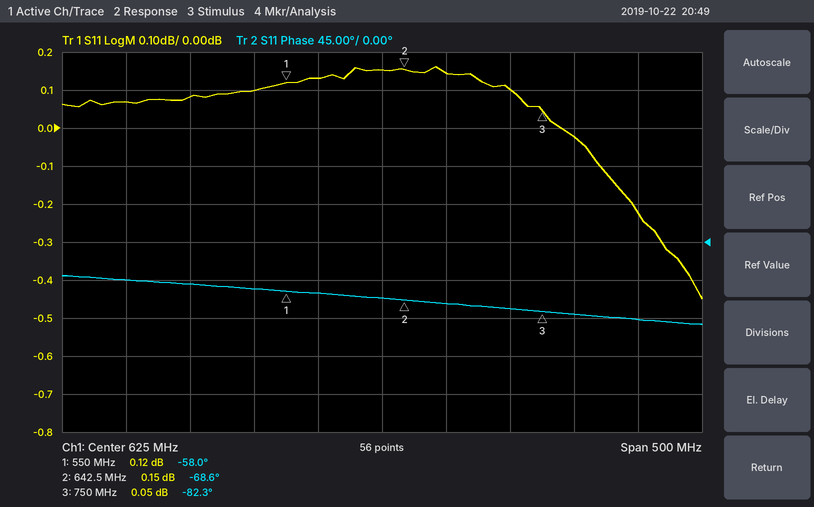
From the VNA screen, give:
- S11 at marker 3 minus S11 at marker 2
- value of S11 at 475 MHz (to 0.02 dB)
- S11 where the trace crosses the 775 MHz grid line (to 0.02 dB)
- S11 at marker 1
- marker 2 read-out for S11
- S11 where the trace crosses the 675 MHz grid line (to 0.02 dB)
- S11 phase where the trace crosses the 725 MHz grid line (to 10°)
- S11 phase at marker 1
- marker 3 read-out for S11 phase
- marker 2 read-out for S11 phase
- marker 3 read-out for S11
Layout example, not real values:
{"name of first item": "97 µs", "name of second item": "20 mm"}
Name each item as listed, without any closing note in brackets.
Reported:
{"S11 at marker 3 minus S11 at marker 2": "-0.10 dB", "value of S11 at 475 MHz": "0.08 dB", "S11 where the trace crosses the 775 MHz grid line": "-0.02 dB", "S11 at marker 1": "0.12 dB", "marker 2 read-out for S11": "0.15 dB", "S11 where the trace crosses the 675 MHz grid line": "0.14 dB", "S11 phase where the trace crosses the 725 MHz grid line": "-80°", "S11 phase at marker 1": "-58.0°", "marker 3 read-out for S11 phase": "-82.3°", "marker 2 read-out for S11 phase": "-68.6°", "marker 3 read-out for S11": "0.05 dB"}
